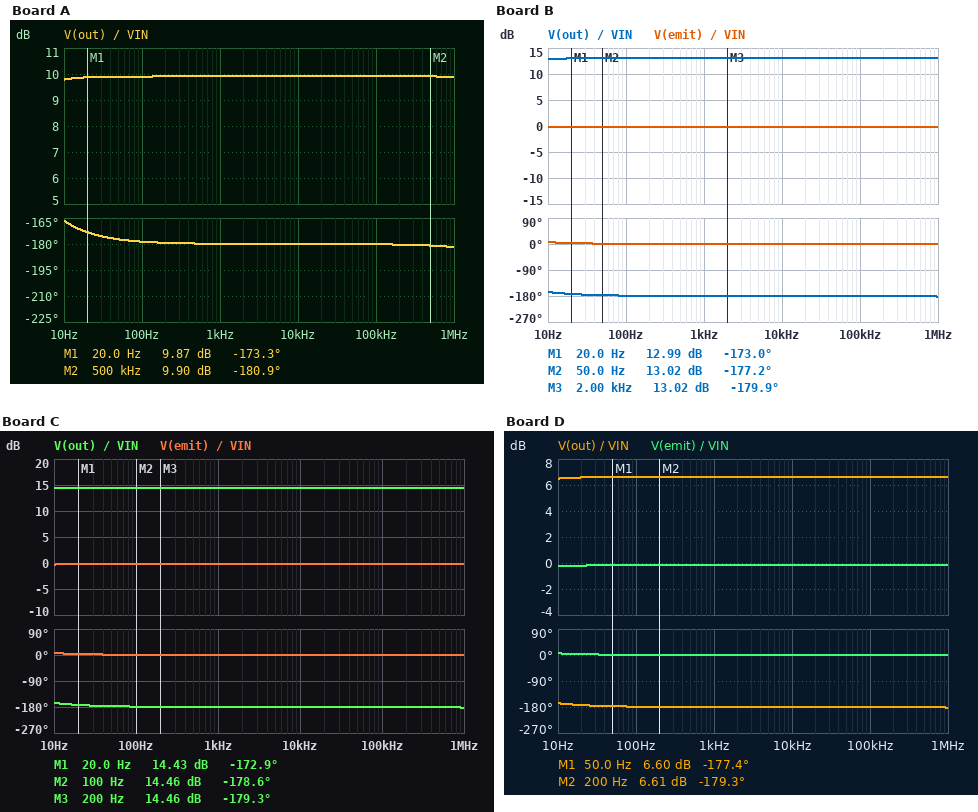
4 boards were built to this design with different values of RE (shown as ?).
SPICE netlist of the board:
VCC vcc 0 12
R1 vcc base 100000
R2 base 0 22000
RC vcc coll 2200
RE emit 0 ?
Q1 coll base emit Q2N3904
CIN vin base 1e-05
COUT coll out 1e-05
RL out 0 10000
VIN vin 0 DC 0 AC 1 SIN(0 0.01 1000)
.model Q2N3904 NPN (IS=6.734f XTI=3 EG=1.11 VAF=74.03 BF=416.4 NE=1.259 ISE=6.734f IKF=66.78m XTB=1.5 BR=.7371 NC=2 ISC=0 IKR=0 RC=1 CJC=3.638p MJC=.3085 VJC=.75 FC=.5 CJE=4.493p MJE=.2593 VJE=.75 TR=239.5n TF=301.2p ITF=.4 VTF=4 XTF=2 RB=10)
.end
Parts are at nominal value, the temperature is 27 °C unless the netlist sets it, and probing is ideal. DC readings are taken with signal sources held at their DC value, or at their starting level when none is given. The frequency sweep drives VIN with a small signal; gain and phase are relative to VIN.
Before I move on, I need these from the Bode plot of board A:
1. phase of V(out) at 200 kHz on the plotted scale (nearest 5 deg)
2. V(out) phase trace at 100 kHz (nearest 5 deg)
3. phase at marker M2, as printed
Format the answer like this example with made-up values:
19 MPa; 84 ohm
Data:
-180 deg; -180 deg; -180.9 deg
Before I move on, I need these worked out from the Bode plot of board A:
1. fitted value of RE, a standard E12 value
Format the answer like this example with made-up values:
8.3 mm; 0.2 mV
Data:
560 Ω
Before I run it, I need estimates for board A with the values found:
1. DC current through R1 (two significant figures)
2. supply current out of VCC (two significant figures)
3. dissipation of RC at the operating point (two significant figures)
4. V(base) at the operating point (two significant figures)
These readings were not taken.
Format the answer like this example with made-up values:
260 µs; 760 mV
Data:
100 µA; 2.3 mA; 10 mW; 1.9 V
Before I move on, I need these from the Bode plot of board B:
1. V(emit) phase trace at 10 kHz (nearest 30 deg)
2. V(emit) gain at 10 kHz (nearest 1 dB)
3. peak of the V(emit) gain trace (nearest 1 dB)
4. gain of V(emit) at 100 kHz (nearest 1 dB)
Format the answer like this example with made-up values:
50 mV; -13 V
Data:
0 deg; 0 dB; 0 dB; 0 dB
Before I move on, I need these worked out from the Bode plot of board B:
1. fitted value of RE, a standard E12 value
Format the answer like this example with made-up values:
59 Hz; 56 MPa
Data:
390 Ω
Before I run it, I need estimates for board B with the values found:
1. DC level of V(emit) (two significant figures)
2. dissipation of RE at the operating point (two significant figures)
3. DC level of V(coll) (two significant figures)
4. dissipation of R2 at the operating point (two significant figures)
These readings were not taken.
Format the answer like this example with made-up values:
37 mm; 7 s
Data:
1.1 V; 3.3 mW; 5.6 V; 150 µW
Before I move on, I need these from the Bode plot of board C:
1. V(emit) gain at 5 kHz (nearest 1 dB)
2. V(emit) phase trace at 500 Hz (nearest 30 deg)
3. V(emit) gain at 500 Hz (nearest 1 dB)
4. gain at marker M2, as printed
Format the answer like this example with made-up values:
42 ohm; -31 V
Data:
0 dB; 0 deg; 0 dB; 14.46 dB
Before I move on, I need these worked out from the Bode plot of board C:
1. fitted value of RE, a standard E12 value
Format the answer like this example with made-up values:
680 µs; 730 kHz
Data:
330 Ω
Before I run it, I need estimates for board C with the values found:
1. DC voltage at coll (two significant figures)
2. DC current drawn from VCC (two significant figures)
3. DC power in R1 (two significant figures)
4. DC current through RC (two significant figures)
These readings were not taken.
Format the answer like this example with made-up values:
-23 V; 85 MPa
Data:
4.8 V; 3.4 mA; 1.0 mW; 3.3 mA
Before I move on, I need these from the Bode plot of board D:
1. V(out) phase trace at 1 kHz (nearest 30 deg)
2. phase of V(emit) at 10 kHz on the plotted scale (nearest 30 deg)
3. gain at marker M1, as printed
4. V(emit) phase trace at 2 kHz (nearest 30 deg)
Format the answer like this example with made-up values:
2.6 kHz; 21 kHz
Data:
-180 deg; 0 deg; 6.60 dB; 0 deg
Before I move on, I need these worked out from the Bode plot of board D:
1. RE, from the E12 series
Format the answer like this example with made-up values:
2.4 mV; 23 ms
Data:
820 Ω
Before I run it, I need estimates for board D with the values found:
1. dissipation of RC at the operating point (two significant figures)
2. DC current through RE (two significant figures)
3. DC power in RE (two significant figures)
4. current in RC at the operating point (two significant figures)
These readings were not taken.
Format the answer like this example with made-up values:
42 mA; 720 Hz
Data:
5.5 mW; 1.6 mA; 2.1 mW; 1.6 mA
